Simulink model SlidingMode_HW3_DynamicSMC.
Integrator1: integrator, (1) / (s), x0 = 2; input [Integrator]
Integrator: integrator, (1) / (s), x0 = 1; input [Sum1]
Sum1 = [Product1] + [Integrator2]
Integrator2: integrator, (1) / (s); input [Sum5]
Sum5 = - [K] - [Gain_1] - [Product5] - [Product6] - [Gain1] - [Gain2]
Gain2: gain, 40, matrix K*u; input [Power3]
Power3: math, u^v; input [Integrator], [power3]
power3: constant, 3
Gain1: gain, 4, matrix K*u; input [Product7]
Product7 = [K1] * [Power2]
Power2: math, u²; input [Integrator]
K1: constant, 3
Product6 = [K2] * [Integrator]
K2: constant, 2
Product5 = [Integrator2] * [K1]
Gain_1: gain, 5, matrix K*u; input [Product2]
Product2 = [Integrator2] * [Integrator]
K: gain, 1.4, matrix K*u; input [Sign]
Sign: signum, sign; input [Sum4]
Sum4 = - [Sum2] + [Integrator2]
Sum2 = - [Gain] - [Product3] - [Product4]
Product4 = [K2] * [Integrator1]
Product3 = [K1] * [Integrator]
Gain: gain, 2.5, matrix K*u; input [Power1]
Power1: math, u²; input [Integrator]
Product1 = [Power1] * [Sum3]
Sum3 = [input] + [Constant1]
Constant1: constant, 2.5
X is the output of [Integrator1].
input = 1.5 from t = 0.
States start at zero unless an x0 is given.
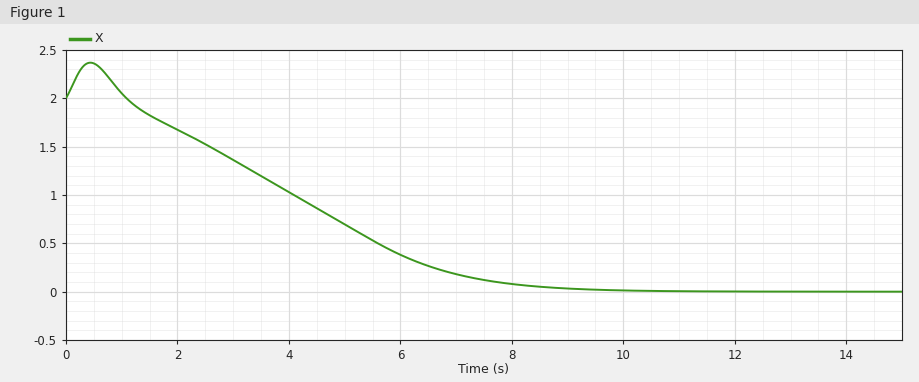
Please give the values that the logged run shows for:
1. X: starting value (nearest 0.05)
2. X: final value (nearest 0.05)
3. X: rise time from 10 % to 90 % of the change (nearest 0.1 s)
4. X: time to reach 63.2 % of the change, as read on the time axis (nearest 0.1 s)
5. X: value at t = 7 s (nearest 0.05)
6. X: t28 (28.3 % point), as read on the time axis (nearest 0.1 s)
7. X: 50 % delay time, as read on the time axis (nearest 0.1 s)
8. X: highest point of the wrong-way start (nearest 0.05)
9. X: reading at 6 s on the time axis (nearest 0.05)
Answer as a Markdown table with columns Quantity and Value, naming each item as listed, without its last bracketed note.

| Quantity | Value |
|---|---|
| X: starting value | 2.00 |
| X: final value | 0.00 |
| X: rise time from 10 % to 90 % of the change | 5.3 s |
| X: time to reach 63.2 % of the change, as read on the time axis | 4.9 s |
| X: value at t = 7 s | 0.20 |
| X: t28 (28.3 % point), as read on the time axis | 2.8 s |
| X: 50 % delay time, as read on the time axis | 4.1 s |
| X: highest point of the wrong-way start | 2.35 |
| X: reading at 6 s on the time axis | 0.40 |
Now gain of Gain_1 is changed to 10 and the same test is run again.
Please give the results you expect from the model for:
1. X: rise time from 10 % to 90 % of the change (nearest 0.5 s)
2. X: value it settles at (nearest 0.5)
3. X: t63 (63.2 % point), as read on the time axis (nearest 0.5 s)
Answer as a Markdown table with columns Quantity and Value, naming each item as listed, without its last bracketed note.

| Quantity | Value |
|---|---|
| X: rise time from 10 % to 90 % of the change | 3.5 s |
| X: value it settles at | 0.0 |
| X: t63 (63.2 % point), as read on the time axis | 9.0 s |
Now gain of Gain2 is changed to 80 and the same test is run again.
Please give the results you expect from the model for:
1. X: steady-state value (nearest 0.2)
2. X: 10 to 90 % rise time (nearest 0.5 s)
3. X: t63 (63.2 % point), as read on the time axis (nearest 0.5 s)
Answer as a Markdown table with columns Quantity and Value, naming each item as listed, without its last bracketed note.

| Quantity | Value |
|---|---|
| X: steady-state value | 0.0 |
| X: 10 to 90 % rise time | 6.5 s |
| X: t63 (63.2 % point), as read on the time axis | 6.0 s |
